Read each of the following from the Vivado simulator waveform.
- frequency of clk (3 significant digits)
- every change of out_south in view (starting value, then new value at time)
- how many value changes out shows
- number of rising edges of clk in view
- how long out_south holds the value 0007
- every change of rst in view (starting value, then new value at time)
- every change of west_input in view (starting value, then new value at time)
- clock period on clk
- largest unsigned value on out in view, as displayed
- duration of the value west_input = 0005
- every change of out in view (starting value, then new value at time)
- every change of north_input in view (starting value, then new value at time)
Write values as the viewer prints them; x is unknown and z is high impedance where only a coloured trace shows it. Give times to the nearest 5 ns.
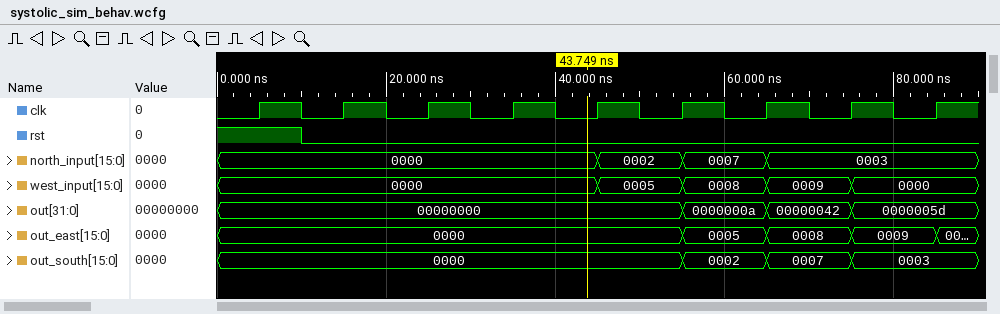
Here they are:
100 MHz
0000, 0002 at 55 ns, 0007 at 65 ns, 0003 at 75 ns
3
9
10 ns
1, 0 at 10 ns
0000, 0005 at 45 ns, 0008 at 55 ns, 0009 at 65 ns, 0000 at 75 ns
10 ns
0000005d
10 ns
00000000, 0000000a at 55 ns, 00000042 at 65 ns, 0000005d at 75 ns
0000, 0002 at 45 ns, 0007 at 55 ns, 0003 at 65 ns
